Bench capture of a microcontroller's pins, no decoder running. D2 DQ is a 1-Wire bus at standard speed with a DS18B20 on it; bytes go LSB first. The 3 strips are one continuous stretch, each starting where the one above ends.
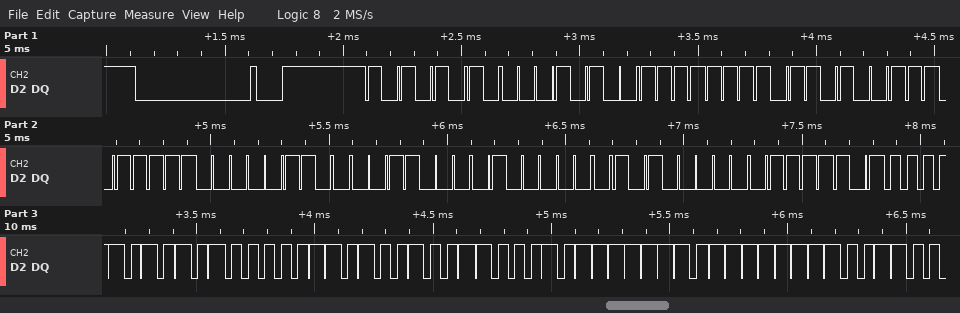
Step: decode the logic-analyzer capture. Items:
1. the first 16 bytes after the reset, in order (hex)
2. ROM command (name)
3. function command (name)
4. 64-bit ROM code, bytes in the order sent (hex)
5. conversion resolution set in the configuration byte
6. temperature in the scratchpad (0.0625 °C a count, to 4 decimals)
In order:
55 28 FF 96 FB 60 18 02 05 BE 50 05 4B 46 7F FF
Match ROM
Read Scratchpad
28 FF 96 FB 60 18 02 05
12 bits
85.0000 °C
